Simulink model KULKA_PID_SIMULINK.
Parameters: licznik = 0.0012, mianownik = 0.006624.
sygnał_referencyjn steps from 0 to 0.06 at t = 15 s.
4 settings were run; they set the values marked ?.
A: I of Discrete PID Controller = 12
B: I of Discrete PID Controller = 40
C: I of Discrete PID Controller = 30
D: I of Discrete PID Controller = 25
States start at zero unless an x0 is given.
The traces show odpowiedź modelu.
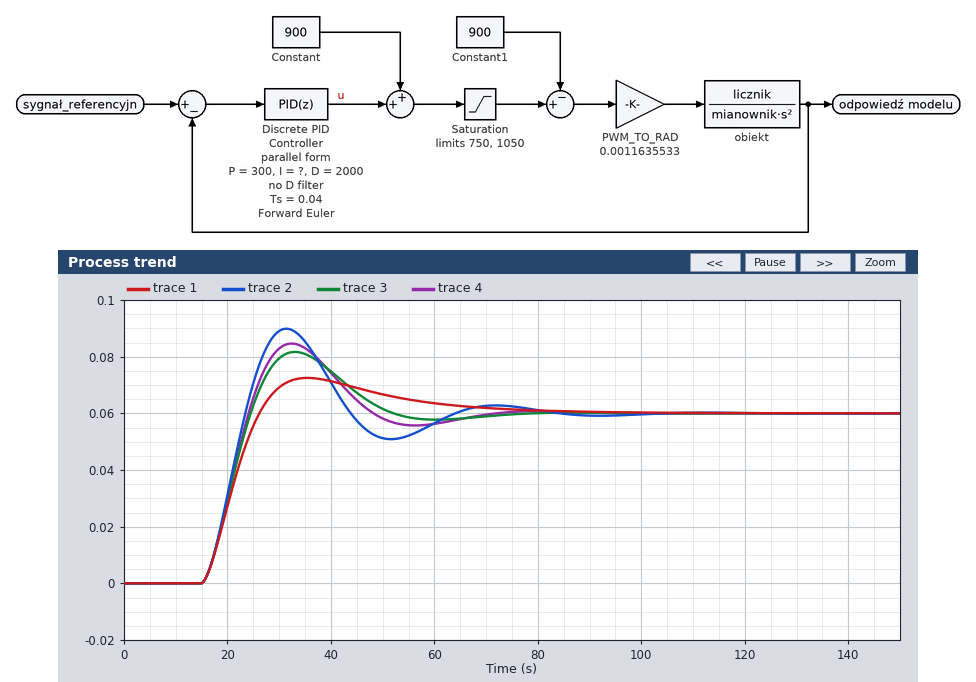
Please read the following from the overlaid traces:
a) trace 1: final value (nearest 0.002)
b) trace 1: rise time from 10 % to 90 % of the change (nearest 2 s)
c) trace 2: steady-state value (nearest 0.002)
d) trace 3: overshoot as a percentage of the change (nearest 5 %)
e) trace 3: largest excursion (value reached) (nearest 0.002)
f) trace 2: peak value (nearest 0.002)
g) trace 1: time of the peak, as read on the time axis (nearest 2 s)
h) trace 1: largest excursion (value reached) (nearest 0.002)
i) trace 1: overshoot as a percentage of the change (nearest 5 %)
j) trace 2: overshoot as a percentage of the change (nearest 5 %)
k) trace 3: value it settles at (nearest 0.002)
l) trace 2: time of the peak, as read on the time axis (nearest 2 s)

0.060
8 s
0.060
35 %
0.082
0.090
36 s
0.072
20 %
50 %
0.060
32 s
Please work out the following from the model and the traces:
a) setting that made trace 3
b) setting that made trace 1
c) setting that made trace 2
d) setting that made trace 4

D
A
B
C
